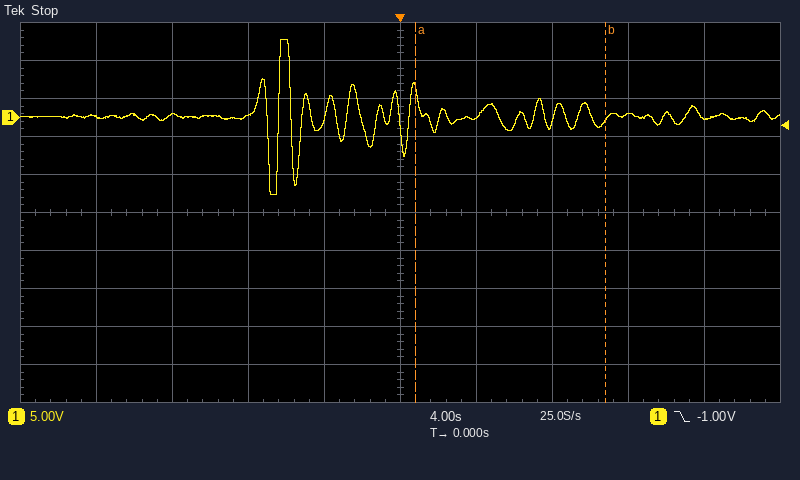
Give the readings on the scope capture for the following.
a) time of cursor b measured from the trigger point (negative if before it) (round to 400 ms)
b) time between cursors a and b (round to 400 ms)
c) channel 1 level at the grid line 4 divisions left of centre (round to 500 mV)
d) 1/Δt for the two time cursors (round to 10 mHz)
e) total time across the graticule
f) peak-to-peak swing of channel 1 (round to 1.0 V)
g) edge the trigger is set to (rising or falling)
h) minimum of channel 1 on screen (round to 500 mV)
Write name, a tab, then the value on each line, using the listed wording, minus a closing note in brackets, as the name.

time of cursor b measured from the trigger point (negative if before it)	+10.8 s
time between cursors a and b	10.0 s
channel 1 level at the grid line 4 divisions left of centre	0.0 V
1/Δt for the two time cursors	100 mHz
total time across the graticule	40 s
peak-to-peak swing of channel 1	20.0 V
edge the trigger is set to	falling
minimum of channel 1 on screen	-10.0 V
